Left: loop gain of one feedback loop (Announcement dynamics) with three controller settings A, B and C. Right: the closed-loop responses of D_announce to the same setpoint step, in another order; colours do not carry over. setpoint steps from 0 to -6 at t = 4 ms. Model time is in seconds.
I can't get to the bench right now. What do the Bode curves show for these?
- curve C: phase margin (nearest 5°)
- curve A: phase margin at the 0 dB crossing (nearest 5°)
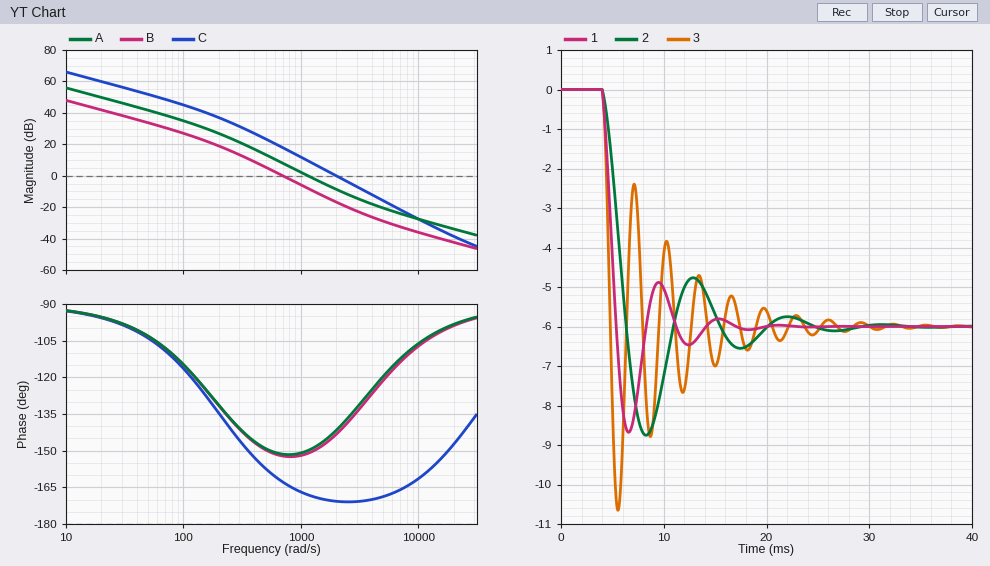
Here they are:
10°
30°
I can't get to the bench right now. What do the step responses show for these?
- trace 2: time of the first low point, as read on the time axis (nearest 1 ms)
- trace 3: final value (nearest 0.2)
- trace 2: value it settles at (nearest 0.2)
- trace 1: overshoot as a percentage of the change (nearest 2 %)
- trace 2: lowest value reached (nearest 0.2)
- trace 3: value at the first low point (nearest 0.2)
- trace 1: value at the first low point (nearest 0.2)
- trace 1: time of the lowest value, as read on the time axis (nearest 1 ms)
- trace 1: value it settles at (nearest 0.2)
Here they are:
8 ms
-6.0
-6.0
44 %
-8.8
-10.6
-8.6
7 ms
-6.0
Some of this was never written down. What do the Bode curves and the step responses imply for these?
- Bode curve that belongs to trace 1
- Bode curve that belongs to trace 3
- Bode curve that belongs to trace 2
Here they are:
A
C
B
